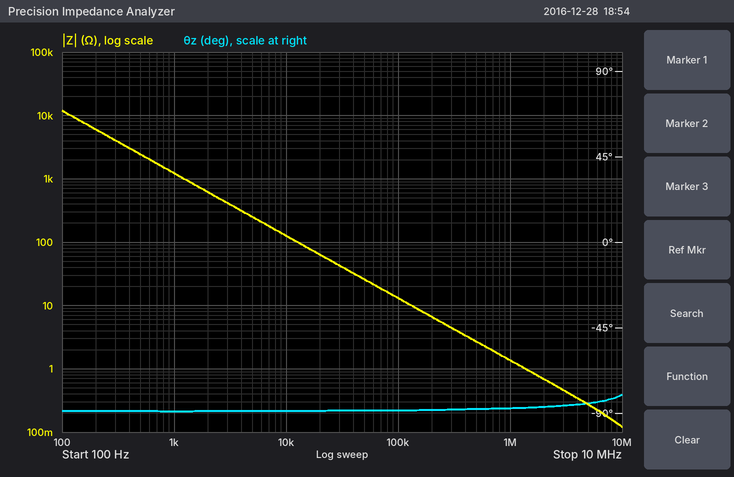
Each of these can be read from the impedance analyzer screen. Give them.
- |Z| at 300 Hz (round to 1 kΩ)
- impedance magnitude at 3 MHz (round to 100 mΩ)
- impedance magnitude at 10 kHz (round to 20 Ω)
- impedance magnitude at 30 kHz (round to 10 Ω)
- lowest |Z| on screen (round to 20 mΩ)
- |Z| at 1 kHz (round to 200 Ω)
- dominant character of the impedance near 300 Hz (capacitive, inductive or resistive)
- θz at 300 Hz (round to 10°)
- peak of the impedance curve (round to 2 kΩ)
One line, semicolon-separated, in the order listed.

4 kΩ; 500 mΩ; 120 Ω; 40 Ω; 120 mΩ; 1.2 kΩ; capacitive; -90°; 12 kΩ
